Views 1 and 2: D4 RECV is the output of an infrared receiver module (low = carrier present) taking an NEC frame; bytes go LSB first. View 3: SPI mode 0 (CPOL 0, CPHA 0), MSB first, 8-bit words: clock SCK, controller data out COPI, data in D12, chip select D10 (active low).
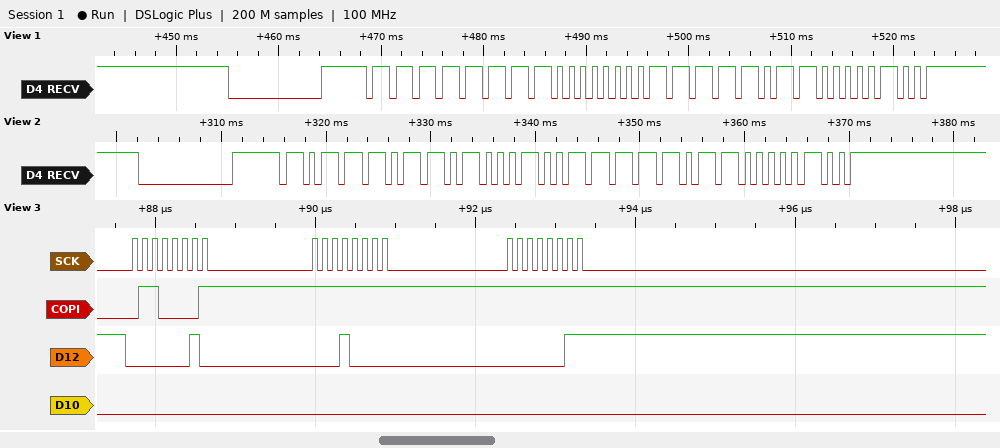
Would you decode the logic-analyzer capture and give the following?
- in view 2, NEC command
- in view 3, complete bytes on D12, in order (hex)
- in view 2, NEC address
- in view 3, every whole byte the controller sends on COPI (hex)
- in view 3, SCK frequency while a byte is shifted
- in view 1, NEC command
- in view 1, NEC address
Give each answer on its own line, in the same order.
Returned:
0xDF
02 10 03
0xDD
61 FF FF
8 MHz
0xDF
0xFF
